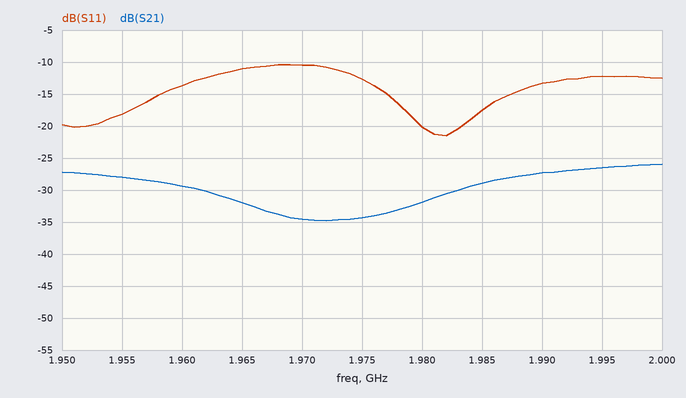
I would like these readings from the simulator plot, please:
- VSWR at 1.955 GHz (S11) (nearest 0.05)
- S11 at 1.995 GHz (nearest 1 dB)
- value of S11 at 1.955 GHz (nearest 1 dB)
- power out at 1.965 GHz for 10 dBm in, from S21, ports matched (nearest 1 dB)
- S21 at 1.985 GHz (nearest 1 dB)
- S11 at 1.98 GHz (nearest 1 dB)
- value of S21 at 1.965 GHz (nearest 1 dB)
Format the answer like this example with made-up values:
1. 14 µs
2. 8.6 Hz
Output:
1. 1.30
2. -12 dB
3. -18 dB
4. -22 dBm
5. -29 dB
6. -20 dB
7. -32 dB
